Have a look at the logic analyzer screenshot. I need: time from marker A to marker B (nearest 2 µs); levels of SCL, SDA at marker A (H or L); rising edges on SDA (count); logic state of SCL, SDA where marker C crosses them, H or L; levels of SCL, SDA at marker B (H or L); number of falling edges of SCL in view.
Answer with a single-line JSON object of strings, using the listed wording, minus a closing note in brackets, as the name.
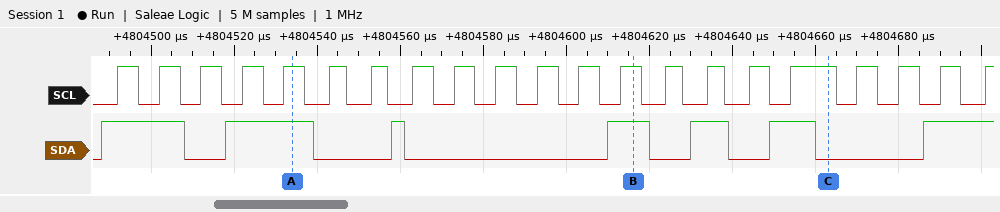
{"time from marker A to marker B": "82 µs", "levels of SCL, SDA at marker A": "SCL=H, SDA=H", "rising edges on SDA": "7", "logic state of SCL, SDA where marker C crosses them, H or L": "SCL=H, SDA=L", "levels of SCL, SDA at marker B": "SCL=H, SDA=H", "number of falling edges of SCL in view": "20"}
